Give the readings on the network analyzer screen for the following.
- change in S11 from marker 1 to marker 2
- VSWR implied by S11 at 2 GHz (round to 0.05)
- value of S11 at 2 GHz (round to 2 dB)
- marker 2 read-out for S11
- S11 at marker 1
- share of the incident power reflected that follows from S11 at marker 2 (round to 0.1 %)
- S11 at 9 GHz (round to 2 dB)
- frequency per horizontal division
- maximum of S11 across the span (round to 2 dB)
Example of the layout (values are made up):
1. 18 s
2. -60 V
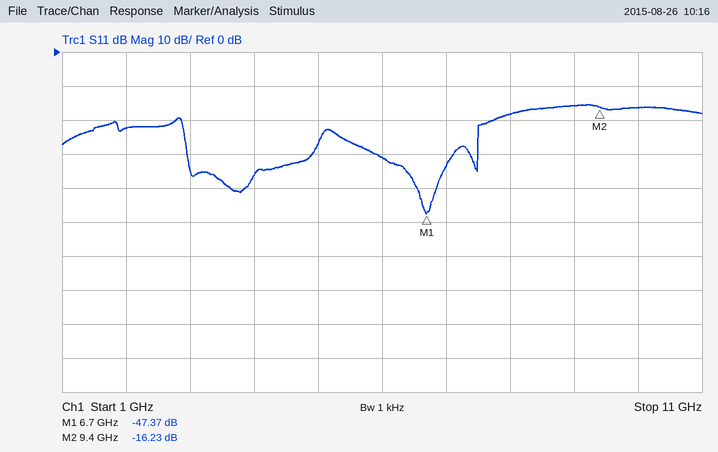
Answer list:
1. 31.14 dB
2. 1.15
3. -22 dB
4. -16.23 dB
5. -47.37 dB
6. 2.4 %
7. -16 dB
8. 1 GHz
9. -16 dB
